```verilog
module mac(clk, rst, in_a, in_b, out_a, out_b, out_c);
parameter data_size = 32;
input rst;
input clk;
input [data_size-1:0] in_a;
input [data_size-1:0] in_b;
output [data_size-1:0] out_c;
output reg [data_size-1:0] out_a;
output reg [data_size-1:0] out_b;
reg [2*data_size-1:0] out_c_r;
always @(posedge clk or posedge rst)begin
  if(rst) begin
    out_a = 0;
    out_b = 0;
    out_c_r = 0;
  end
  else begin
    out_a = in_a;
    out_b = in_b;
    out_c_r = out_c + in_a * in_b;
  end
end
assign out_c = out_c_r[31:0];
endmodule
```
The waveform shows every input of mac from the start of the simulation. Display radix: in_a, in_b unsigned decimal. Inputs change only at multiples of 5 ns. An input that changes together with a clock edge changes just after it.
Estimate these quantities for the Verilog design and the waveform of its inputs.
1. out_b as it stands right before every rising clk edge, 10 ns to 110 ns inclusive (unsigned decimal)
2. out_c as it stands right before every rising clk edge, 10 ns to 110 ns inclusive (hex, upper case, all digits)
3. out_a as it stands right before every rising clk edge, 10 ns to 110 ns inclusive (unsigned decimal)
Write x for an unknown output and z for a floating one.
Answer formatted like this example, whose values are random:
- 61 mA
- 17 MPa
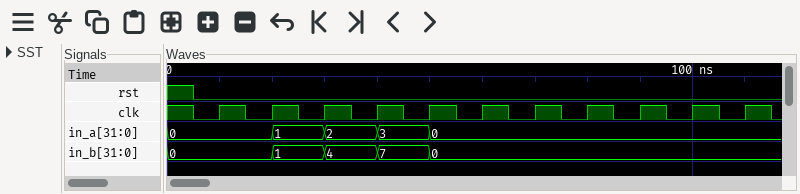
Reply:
- 0, 0, 0, 1, 4, 7, 0, 0, 0, 0, 0
- 00000000, 00000000, 00000000, 00000001, 00000009, 0000001E, 0000001E, 0000001E, 0000001E, 0000001E, 0000001E
- 0, 0, 0, 1, 2, 3, 0, 0, 0, 0, 0
